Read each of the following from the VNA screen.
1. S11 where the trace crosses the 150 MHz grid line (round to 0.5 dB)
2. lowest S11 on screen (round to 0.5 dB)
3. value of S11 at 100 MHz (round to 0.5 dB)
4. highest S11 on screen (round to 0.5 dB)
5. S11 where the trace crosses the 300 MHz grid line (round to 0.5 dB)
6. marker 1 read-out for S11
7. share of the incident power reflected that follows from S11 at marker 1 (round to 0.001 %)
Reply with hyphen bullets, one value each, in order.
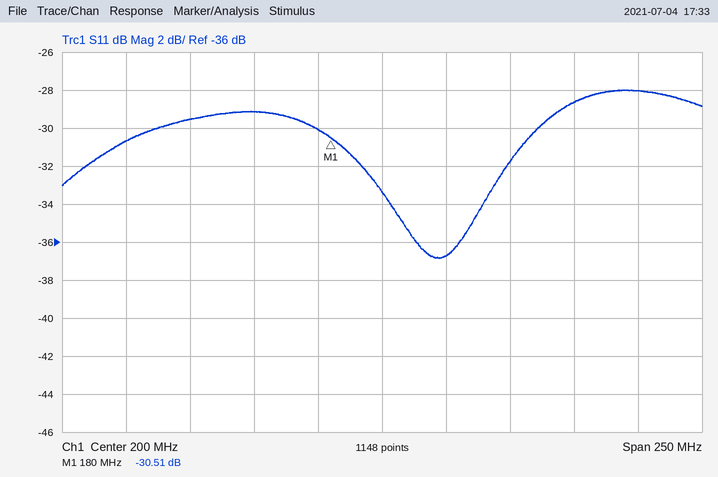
- -29.0 dB
- -37.0 dB
- -30.5 dB
- -28.0 dB
- -28.0 dB
- -30.51 dB
- 0.089 %
